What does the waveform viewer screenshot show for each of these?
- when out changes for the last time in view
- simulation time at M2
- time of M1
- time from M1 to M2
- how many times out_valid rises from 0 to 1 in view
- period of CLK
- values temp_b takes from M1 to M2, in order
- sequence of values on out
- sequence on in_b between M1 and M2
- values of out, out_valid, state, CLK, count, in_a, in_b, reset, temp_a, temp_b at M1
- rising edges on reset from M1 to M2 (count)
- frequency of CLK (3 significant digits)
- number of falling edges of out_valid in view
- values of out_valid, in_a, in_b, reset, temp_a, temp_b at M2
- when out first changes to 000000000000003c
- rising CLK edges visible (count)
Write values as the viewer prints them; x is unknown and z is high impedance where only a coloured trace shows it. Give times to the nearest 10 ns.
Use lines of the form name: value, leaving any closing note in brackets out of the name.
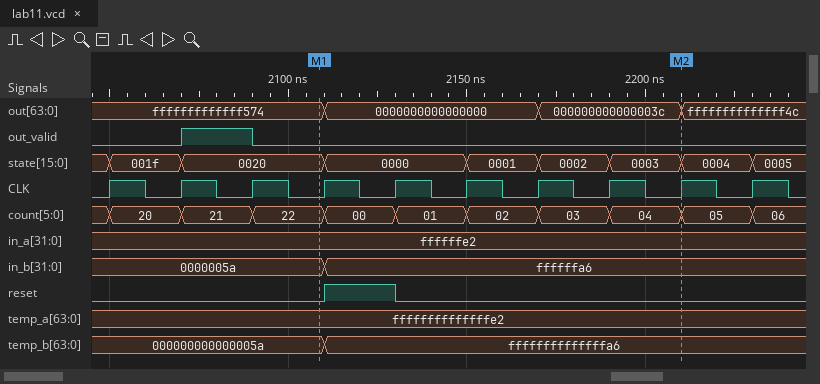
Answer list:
when out changes for the last time in view: 2210 ns
simulation time at M2: 2210 ns
time of M1: 2110 ns
time from M1 to M2: 100 ns
how many times out_valid rises from 0 to 1 in view: 1
period of CLK: 20 ns
values temp_b takes from M1 to M2, in order: 000000000000005a, ffffffffffffffa6
sequence of values on out: fffffffffffff574, 0000000000000000, 000000000000003c, ffffffffffffff4c
sequence on in_b between M1 and M2: 0000005a, ffffffa6
values of out, out_valid, state, CLK, count, in_a, in_b, reset, temp_a, temp_b at M1: out=fffffffffffff574, out_valid=0, state=0020, CLK=0, count=22, in_a=ffffffe2, in_b=0000005a, reset=0, temp_a=ffffffffffffffe2, temp_b=000000000000005a
rising edges on reset from M1 to M2: 1
frequency of CLK: 50.0 MHz
number of falling edges of out_valid in view: 1
values of out_valid, in_a, in_b, reset, temp_a, temp_b at M2: out_valid=0, in_a=ffffffe2, in_b=ffffffa6, reset=0, temp_a=ffffffffffffffe2, temp_b=ffffffffffffffa6
when out first changes to 000000000000003c: 2170 ns
rising CLK edges visible: 10
